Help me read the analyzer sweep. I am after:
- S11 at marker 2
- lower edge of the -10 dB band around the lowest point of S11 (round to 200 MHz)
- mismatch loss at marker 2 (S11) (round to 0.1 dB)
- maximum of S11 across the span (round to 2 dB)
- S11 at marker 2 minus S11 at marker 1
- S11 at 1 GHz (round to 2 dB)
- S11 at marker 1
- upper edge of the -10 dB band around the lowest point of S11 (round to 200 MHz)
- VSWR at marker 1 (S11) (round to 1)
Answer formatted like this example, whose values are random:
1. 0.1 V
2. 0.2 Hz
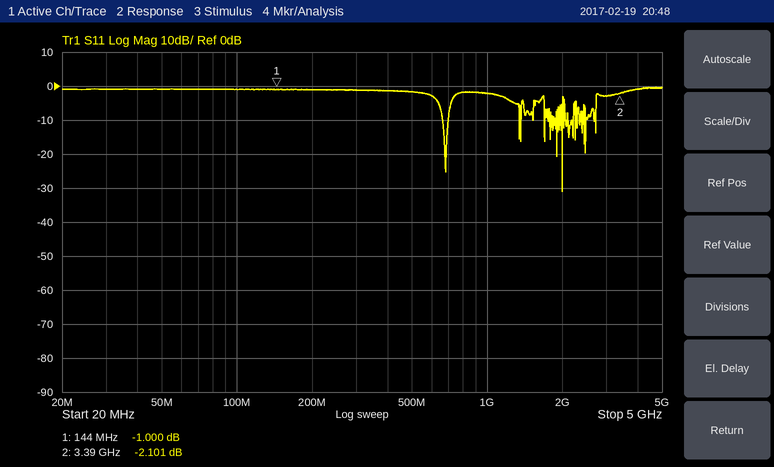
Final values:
1. -2.101 dB
2. 2.0 GHz
3. 4.2 dB
4. 0 dB
5. -1.101 dB
6. -2 dB
7. -1.000 dB
8. 2.0 GHz
9. 17
